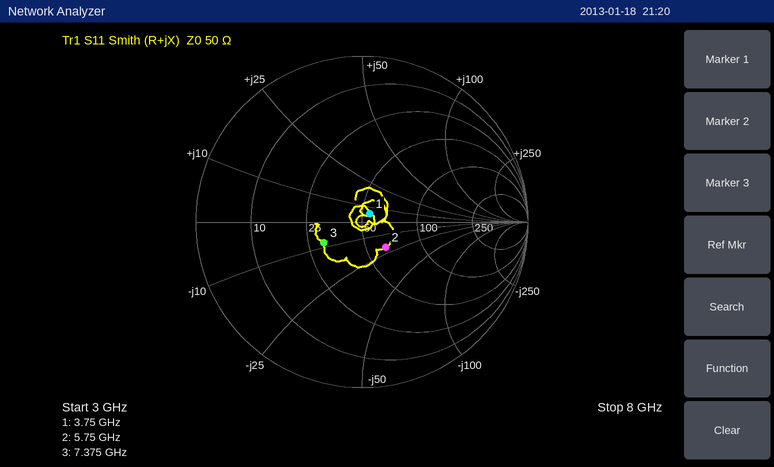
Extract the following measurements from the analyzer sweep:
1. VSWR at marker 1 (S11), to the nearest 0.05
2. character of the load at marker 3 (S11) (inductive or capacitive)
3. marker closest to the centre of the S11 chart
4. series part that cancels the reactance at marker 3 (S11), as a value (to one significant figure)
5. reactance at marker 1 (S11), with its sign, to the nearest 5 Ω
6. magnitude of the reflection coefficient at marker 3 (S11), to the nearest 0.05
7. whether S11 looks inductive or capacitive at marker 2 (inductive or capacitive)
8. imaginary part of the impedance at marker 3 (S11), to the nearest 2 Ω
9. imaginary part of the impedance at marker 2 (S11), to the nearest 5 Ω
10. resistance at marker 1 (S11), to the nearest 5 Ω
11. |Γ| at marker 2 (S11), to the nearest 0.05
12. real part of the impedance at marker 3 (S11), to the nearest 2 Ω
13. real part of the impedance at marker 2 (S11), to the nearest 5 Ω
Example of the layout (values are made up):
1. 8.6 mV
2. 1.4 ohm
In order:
1. 1.15
2. capacitive
3. marker 1
4. 200 pH
5. +5 Ω
6. 0.25
7. capacitive
8. -8 Ω
9. -20 Ω
10. 55 Ω
11. 0.20
12. 30 Ω
13. 65 Ω
